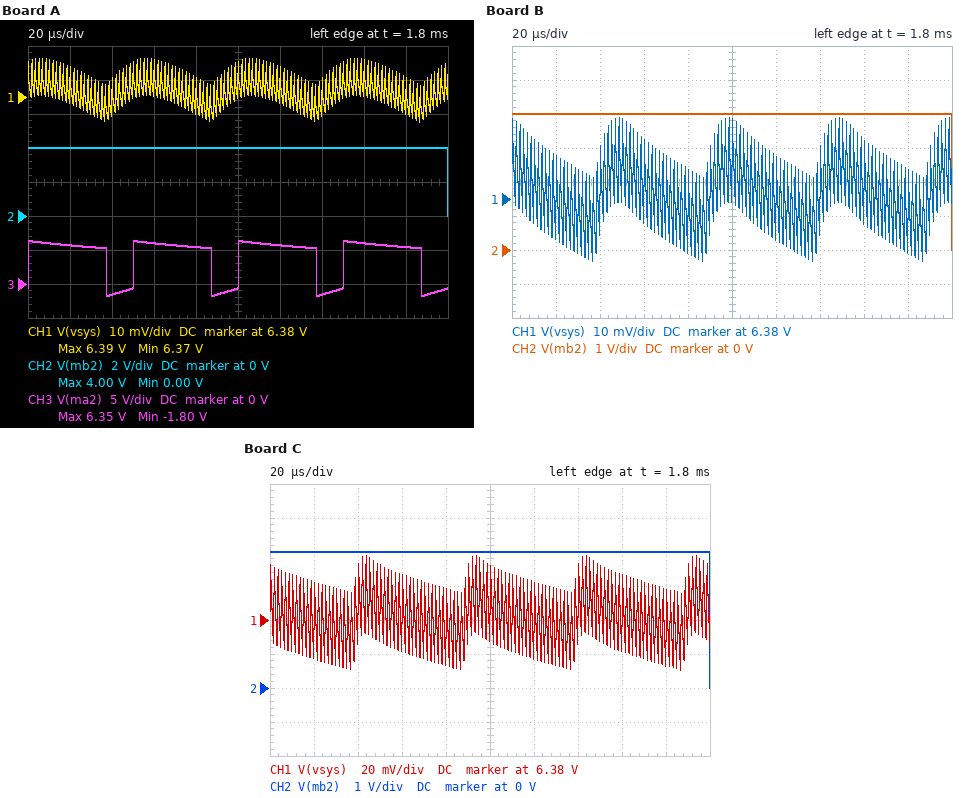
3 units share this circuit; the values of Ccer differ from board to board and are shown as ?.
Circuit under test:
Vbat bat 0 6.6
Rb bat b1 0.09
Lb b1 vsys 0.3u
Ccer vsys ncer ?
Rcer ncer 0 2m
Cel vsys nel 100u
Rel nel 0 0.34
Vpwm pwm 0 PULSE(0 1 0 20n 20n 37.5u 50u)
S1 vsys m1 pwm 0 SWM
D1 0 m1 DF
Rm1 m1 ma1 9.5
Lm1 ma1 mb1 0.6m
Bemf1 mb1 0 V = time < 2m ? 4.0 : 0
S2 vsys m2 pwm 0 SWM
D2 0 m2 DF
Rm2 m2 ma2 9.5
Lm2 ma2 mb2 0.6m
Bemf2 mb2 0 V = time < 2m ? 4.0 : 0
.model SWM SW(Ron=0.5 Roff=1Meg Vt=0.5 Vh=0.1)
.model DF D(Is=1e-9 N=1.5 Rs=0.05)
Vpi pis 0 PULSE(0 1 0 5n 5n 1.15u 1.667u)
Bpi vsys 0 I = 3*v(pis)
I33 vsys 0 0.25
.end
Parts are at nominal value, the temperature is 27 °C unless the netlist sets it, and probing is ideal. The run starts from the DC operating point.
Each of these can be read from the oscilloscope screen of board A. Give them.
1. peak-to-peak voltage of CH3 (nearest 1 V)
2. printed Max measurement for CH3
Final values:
8 V
6.35 V
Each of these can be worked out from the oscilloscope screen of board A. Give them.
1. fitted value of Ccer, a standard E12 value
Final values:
220 µF
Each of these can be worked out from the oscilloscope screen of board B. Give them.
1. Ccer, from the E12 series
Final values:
56 µF
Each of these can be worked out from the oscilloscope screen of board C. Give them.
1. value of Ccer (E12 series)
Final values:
27 µF
